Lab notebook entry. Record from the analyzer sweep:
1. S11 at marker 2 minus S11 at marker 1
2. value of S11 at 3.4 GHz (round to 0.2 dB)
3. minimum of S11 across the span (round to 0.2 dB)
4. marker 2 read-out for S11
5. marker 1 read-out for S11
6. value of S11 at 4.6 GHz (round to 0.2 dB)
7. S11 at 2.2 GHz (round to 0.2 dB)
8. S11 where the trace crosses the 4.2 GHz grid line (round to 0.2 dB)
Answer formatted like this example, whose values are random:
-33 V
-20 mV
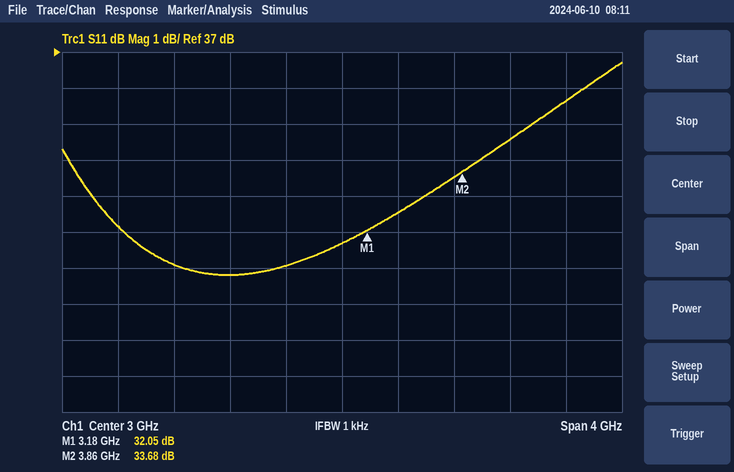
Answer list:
1.63 dB
32.6 dB
30.8 dB
33.68 dB
32.05 dB
35.6 dB
30.8 dB
34.6 dB
